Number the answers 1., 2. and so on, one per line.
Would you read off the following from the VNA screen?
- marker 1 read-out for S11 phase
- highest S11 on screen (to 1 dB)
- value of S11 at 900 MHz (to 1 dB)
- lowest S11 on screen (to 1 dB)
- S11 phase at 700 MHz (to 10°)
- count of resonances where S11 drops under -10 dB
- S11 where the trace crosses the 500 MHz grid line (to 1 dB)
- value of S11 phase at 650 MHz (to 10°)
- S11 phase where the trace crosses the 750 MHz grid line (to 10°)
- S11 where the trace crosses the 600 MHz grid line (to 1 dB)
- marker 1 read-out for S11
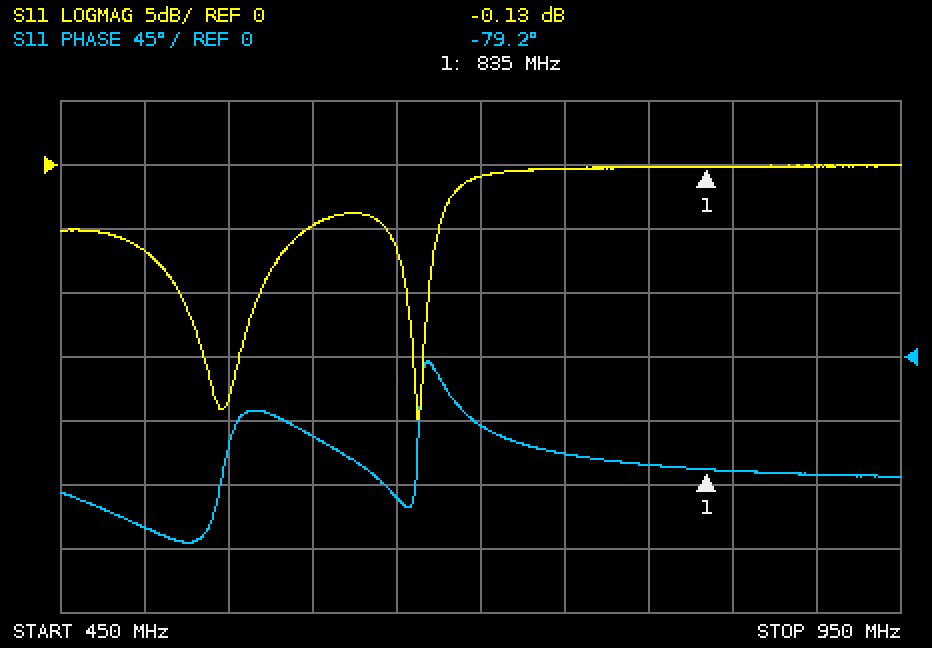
1. -79.2°
2. 0 dB
3. 0 dB
4. -20 dB
5. -50°
6. 2
7. -7 dB
8. -100°
9. -70°
10. -5 dB
11. -0.13 dB
